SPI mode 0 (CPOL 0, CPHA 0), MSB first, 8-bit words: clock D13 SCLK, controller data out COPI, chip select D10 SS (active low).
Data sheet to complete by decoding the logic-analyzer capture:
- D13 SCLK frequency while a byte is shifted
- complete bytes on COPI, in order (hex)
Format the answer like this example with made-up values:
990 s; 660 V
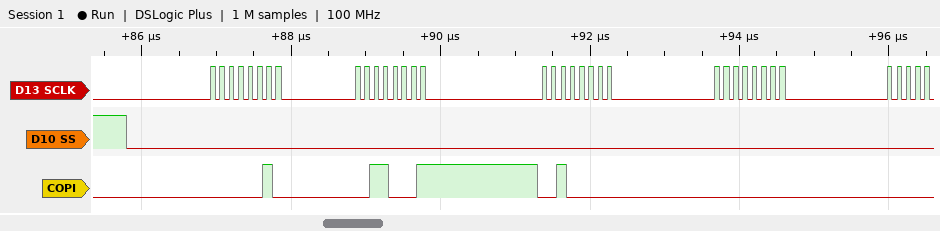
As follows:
8 MHz; 02 31 20 00
